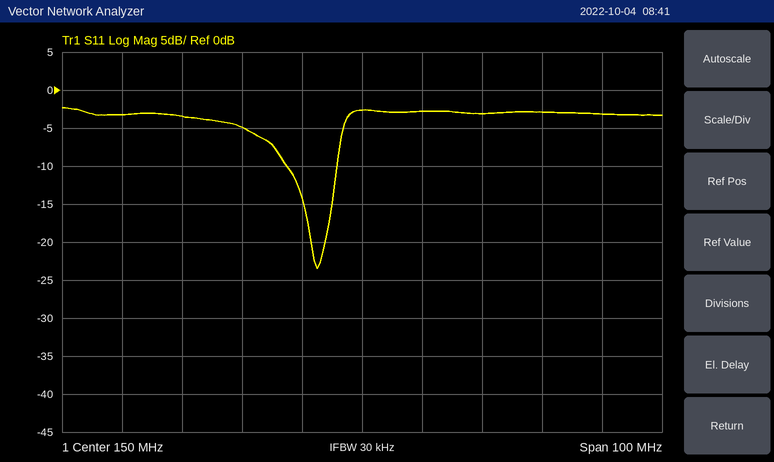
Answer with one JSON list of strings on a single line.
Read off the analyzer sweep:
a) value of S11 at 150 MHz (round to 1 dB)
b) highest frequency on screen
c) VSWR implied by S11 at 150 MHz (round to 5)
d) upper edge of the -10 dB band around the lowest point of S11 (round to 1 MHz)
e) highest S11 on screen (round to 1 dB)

["-3 dB", "200 MHz", "5", "146 MHz", "-2 dB"]
